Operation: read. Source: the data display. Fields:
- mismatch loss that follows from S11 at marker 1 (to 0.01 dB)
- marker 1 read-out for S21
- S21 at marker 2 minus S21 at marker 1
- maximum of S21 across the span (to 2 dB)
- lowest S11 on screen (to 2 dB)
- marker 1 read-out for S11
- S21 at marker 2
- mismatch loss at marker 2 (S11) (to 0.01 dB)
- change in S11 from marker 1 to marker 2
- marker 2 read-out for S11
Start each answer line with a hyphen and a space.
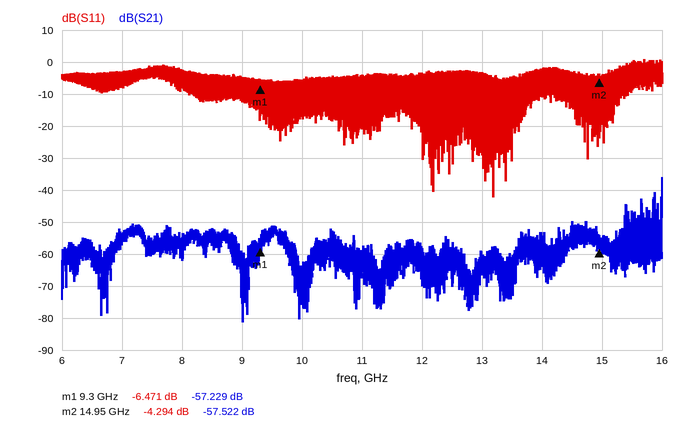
- 1.11 dB
- -57.229 dB
- -0.293 dB
- -36 dB
- -42 dB
- -6.471 dB
- -57.522 dB
- 2.02 dB
- 2.177 dB
- -4.294 dB
